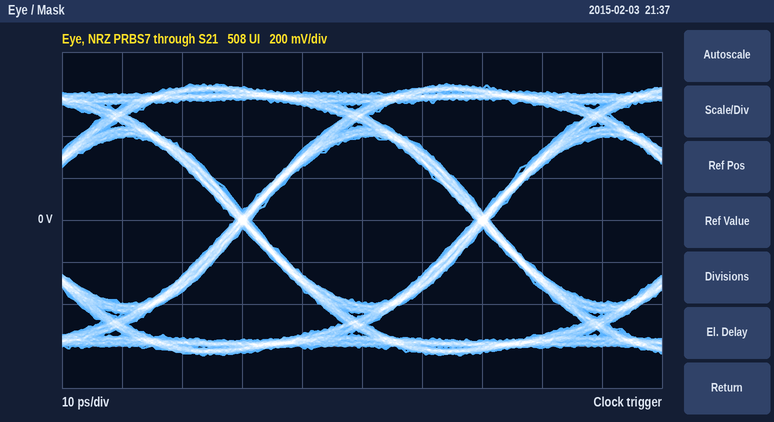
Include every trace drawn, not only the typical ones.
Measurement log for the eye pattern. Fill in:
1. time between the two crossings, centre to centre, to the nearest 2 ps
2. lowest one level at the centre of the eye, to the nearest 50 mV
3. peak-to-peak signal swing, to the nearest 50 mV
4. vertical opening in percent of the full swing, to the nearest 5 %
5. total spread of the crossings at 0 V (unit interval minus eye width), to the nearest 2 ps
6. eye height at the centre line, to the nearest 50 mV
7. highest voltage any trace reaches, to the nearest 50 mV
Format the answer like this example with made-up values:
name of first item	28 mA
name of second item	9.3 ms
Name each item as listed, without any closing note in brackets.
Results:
time between the two crossings, centre to centre, to the nearest 2 ps	40 ps
lowest one level at the centre of the eye, to the nearest 50 mV	400 mV
peak-to-peak signal swing, to the nearest 50 mV	1.30 V
vertical opening in percent of the full swing, to the nearest 5 %	60 %
total spread of the crossings at 0 V (unit interval minus eye width), to the nearest 2 ps	2 ps
eye height at the centre line, to the nearest 50 mV	800 mV
highest voltage any trace reaches, to the nearest 50 mV	650 mV
